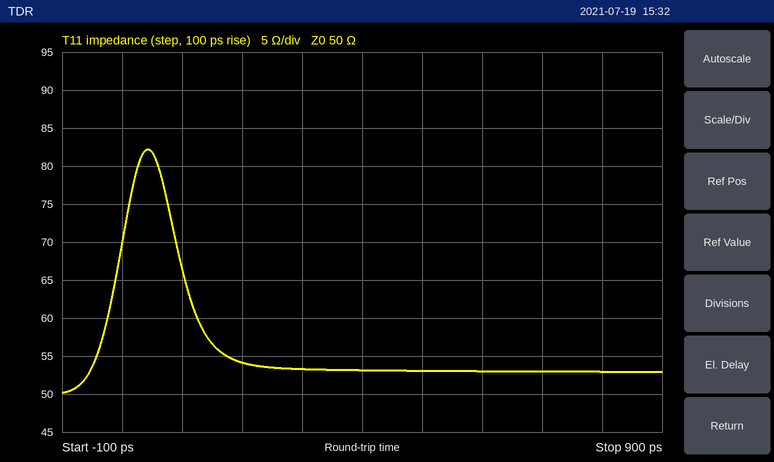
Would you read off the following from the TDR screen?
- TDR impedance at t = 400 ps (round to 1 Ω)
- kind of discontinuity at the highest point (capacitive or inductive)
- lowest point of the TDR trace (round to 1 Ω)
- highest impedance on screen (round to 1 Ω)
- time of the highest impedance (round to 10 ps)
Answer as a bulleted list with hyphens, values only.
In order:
- 53 Ω
- inductive
- 50 Ω
- 82 Ω
- 40 ps
